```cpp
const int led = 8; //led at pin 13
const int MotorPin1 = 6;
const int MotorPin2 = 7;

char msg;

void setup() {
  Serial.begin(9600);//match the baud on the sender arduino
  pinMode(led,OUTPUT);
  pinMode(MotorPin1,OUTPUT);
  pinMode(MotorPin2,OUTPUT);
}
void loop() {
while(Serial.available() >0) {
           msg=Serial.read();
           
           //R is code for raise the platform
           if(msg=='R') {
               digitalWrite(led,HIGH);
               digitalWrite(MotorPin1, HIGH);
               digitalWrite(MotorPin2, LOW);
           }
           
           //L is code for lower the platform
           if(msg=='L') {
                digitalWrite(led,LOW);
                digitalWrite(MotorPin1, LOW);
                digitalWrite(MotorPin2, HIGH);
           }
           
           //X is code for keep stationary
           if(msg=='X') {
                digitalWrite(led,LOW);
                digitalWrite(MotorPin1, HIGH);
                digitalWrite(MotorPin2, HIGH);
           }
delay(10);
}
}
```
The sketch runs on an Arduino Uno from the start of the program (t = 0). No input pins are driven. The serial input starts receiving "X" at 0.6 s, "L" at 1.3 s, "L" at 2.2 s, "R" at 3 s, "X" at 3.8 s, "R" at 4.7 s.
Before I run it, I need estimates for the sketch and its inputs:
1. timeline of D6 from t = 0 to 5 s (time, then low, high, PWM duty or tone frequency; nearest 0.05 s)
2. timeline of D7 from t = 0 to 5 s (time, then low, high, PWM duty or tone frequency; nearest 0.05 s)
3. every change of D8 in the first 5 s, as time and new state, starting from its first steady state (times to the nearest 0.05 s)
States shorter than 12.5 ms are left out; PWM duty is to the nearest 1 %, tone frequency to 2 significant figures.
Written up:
0 s low; 0.6 s high; 1.3 s low; 3 s high
0 s low; 0.6 s high; 3 s low; 3.8 s high; 4.7 s low
0 s low; 3 s high; 3.8 s low; 4.7 s high
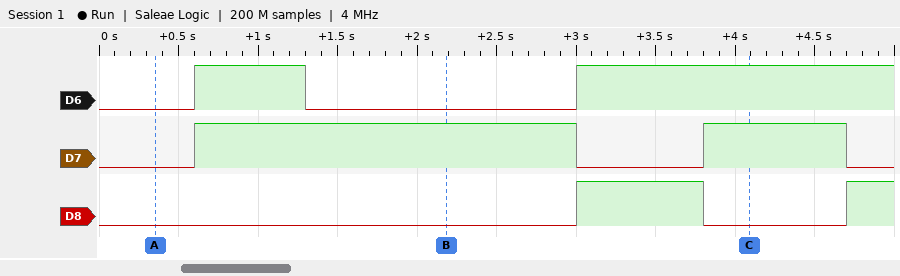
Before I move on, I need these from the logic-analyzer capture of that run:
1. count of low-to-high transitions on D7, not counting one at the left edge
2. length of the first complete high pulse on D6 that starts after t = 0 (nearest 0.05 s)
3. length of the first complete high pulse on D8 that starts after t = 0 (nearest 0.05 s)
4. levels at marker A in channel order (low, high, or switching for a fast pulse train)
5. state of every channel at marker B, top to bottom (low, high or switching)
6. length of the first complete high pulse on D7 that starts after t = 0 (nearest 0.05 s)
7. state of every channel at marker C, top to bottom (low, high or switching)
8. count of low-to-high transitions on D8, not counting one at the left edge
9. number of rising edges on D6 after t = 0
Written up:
2
0.70 s
0.80 s
D6 low, D7 low, D8 low
D6 low, D7 high, D8 low
2.40 s
D6 high, D7 high, D8 low
2
2
